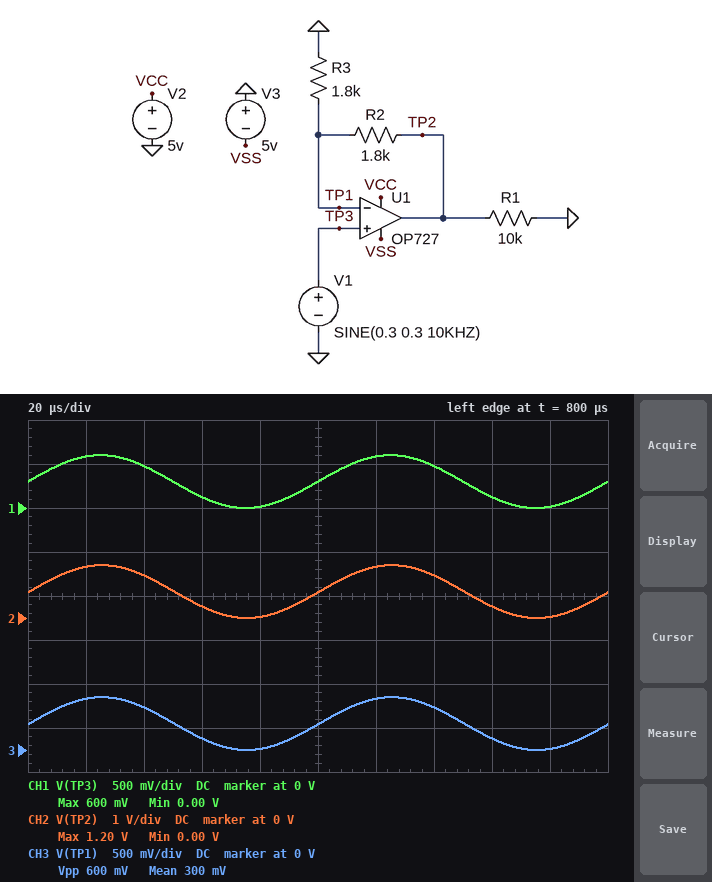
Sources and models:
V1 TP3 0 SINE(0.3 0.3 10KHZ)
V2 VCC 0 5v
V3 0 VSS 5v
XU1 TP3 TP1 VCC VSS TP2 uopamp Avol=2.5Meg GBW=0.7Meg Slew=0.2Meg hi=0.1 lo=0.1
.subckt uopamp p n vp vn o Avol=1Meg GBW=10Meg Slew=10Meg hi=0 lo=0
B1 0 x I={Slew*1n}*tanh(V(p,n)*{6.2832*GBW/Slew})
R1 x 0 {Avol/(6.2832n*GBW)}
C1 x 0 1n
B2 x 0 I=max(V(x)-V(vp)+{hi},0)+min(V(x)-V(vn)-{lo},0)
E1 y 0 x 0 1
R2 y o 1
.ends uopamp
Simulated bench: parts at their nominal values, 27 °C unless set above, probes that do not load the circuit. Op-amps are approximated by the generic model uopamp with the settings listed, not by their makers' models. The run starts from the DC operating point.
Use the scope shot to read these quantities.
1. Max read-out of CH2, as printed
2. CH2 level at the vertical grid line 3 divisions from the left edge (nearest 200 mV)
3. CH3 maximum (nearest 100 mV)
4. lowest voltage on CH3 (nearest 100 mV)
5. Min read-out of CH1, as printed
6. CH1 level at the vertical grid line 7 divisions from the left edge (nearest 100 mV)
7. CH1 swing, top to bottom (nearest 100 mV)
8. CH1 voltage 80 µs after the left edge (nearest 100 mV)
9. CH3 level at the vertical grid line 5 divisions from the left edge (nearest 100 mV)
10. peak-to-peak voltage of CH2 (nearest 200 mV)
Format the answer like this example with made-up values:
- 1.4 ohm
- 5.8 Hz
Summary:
- 1.20 V
- 200 mV
- 600 mV
- 0 V
- 0.00 V
- 500 mV
- 600 mV
- 0 V
- 300 mV
- 1.2 V
